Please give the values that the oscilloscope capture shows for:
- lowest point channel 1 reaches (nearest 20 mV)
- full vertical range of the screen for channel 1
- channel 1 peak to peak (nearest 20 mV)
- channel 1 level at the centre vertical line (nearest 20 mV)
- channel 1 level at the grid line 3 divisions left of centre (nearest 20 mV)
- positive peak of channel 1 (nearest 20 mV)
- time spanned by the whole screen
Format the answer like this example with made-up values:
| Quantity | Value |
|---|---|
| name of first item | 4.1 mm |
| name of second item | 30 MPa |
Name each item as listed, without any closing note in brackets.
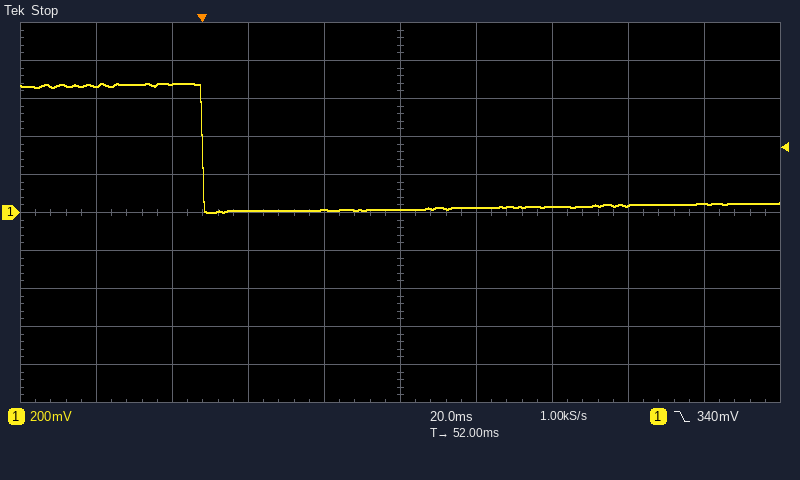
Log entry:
| Quantity | Value |
|---|---|
| lowest point channel 1 reaches | 0 mV |
| full vertical range of the screen for channel 1 | 2 V |
| channel 1 peak to peak | 680 mV |
| channel 1 level at the centre vertical line | 20 mV |
| channel 1 level at the grid line 3 divisions left of centre | 680 mV |
| positive peak of channel 1 | 680 mV |
| time spanned by the whole screen | 200 ms |
